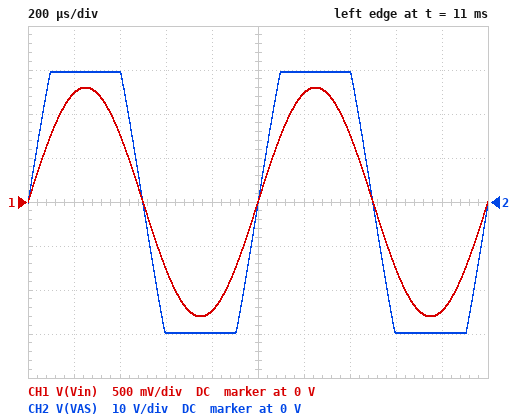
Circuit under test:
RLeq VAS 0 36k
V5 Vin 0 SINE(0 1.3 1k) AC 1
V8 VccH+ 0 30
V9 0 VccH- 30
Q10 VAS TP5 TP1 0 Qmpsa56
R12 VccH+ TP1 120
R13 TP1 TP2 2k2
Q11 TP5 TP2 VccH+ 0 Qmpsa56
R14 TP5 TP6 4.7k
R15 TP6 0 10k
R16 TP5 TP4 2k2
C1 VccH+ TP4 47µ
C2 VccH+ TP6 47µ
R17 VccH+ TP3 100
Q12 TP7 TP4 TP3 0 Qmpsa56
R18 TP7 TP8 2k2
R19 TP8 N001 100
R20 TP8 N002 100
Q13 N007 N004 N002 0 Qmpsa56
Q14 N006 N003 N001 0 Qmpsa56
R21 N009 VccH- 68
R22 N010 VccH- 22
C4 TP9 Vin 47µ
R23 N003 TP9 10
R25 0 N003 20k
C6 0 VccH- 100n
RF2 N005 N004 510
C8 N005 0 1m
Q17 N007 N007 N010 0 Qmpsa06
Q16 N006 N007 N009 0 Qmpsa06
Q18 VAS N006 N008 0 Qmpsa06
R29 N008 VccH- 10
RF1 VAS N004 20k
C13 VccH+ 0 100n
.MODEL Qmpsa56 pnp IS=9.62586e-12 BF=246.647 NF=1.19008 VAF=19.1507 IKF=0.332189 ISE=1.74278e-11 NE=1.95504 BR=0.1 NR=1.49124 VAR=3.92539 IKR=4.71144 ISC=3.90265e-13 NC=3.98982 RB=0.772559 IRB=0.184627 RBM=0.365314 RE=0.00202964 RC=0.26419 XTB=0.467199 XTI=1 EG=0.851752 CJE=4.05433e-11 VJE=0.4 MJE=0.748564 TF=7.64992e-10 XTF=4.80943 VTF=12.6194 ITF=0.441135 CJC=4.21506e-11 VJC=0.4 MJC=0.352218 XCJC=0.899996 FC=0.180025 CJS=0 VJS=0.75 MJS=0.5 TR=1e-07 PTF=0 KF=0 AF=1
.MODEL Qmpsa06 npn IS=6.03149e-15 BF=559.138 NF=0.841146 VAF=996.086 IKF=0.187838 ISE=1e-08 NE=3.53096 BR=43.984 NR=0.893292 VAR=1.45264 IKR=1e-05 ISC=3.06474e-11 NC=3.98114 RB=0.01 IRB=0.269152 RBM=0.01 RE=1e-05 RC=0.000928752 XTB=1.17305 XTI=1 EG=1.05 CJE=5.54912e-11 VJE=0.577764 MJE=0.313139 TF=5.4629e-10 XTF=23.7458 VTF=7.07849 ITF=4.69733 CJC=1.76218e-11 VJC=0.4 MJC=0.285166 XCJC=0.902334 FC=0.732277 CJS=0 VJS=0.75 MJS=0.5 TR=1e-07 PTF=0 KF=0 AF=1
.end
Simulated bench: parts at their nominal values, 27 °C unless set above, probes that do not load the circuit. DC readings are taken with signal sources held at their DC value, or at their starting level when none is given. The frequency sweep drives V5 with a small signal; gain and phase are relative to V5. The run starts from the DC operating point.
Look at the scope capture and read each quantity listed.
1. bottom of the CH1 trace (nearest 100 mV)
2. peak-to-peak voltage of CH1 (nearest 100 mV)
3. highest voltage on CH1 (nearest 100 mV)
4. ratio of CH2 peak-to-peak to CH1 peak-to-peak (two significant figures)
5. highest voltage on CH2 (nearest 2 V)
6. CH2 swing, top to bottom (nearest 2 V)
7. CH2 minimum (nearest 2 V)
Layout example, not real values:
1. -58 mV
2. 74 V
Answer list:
1. -1.3 V
2. 2.6 V
3. 1.3 V
4. 23
5. 30 V
6. 60 V
7. -30 V
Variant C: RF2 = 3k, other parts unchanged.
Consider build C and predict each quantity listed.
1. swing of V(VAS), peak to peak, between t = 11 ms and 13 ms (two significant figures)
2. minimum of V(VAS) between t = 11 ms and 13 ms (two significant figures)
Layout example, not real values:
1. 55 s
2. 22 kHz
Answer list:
1. 20 V
2. -10 V
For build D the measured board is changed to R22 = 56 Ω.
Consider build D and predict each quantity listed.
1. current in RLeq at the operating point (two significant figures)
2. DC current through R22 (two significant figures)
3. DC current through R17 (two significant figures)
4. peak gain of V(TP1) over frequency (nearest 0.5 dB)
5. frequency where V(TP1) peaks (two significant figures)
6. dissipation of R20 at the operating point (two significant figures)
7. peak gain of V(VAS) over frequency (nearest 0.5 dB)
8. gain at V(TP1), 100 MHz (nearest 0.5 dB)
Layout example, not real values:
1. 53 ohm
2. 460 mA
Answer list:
1. 2.1 µA
2. 3.0 mA
3. 5.7 mA
4. 5.0 dB
5. 7.6 MHz
6. 940 µW
7. 34.0 dB
8. -15.0 dB
